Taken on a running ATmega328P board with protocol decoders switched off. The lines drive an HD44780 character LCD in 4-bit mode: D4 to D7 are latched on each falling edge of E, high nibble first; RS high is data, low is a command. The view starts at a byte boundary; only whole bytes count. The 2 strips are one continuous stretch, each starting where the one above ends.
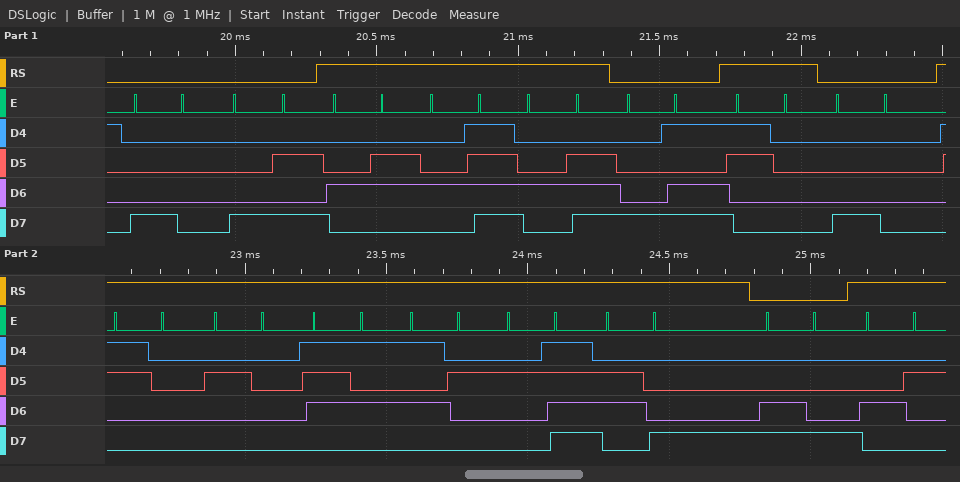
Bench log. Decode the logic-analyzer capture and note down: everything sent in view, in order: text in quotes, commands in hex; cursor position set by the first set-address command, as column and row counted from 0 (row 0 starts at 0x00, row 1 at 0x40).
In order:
0x80 0x8A "FON" 0x8D "0" 0x80 "0 uR/h" 0xC8 "B"
column 0, row 0
